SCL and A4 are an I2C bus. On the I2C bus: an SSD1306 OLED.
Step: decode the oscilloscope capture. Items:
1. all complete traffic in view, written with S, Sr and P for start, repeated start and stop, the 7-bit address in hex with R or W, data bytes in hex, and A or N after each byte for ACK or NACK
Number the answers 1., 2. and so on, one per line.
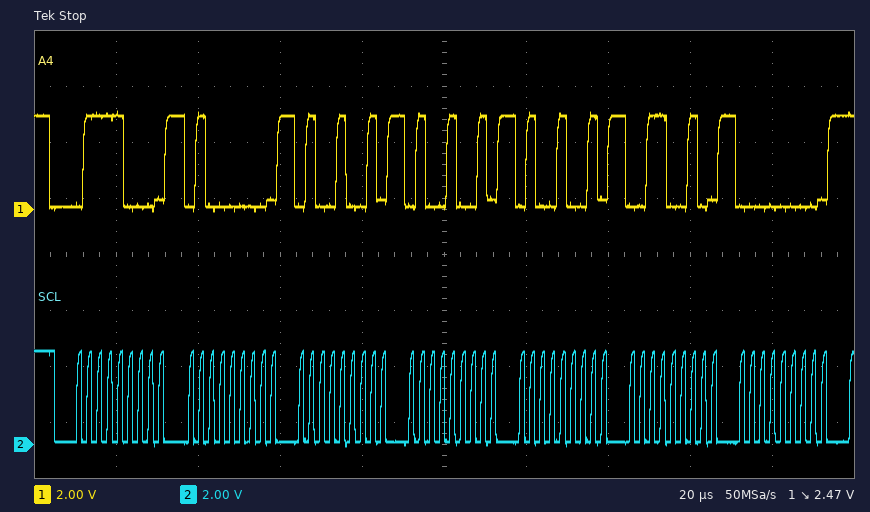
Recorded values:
1. S 3CW A 40 A 49 A 49 A 49 A 32 A 00 A
